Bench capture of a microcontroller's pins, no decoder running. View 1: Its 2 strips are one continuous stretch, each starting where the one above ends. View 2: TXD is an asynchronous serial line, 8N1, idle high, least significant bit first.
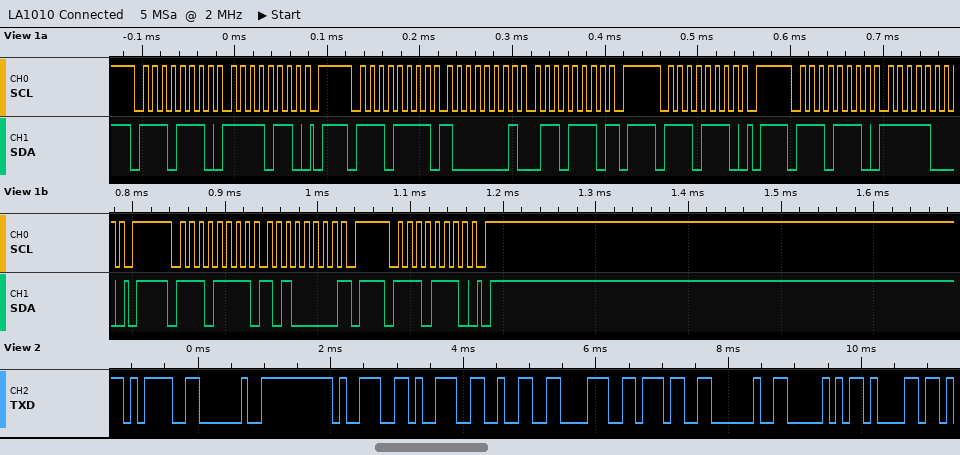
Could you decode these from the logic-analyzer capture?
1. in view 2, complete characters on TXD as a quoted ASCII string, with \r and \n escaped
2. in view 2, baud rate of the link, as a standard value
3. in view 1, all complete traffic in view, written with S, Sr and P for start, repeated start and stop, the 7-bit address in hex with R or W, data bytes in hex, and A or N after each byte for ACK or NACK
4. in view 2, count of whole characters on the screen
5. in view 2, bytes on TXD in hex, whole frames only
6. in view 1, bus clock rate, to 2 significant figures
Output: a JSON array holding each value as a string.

["\"= 99287 Pa\"", "9600 baud", "S 77W A F6 A P S 77R A 81 A 6E N P S 77W A P S 77W A F8 A P S 77R A A0 N P S 77W A P", "10", "0x3D 0x20 0x39 0x39 0x32 0x38 0x37 0x20 0x50 0x61", "100 kHz"]
